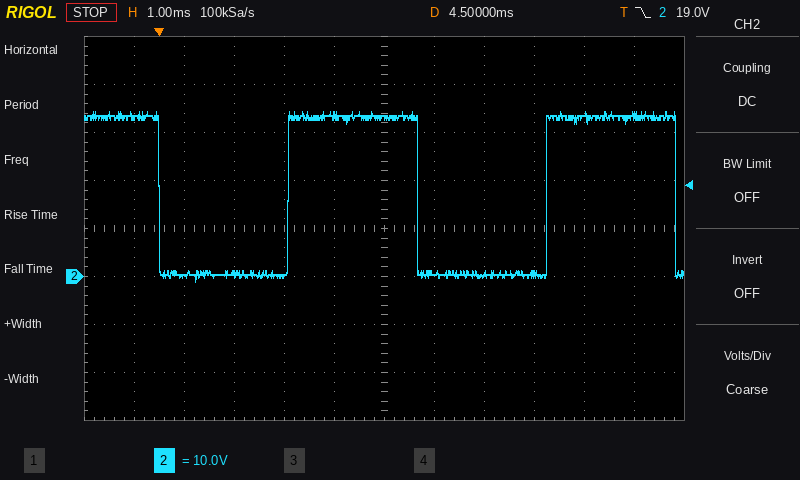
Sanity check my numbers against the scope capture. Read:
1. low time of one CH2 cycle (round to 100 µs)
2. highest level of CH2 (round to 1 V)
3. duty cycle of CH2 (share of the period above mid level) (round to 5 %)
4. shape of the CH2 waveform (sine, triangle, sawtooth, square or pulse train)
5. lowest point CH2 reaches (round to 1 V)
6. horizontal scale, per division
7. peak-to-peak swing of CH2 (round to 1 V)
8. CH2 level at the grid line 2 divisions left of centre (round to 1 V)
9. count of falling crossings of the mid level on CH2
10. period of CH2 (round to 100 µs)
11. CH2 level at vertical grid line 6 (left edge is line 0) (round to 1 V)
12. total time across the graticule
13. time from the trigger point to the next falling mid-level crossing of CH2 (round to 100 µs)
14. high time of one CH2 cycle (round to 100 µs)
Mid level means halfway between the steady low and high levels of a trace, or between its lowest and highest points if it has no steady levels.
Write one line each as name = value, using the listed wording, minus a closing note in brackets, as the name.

low time of one CH2 cycle = 2.6 ms
highest level of CH2 = 34 V
duty cycle of CH2 (share of the period above mid level) = 50 %
shape of the CH2 waveform = square
lowest point CH2 reaches = -1 V
horizontal scale, per division = 1 ms
peak-to-peak swing of CH2 = 35 V
CH2 level at the grid line 2 divisions left of centre = 0 V
count of falling crossings of the mid level on CH2 = 3
period of CH2 = 5.2 ms
CH2 level at vertical grid line 6 (left edge is line 0) = 33 V
total time across the graticule = 12 ms
time from the trigger point to the next falling mid-level crossing of CH2 = 5.2 ms
high time of one CH2 cycle = 2.6 ms
